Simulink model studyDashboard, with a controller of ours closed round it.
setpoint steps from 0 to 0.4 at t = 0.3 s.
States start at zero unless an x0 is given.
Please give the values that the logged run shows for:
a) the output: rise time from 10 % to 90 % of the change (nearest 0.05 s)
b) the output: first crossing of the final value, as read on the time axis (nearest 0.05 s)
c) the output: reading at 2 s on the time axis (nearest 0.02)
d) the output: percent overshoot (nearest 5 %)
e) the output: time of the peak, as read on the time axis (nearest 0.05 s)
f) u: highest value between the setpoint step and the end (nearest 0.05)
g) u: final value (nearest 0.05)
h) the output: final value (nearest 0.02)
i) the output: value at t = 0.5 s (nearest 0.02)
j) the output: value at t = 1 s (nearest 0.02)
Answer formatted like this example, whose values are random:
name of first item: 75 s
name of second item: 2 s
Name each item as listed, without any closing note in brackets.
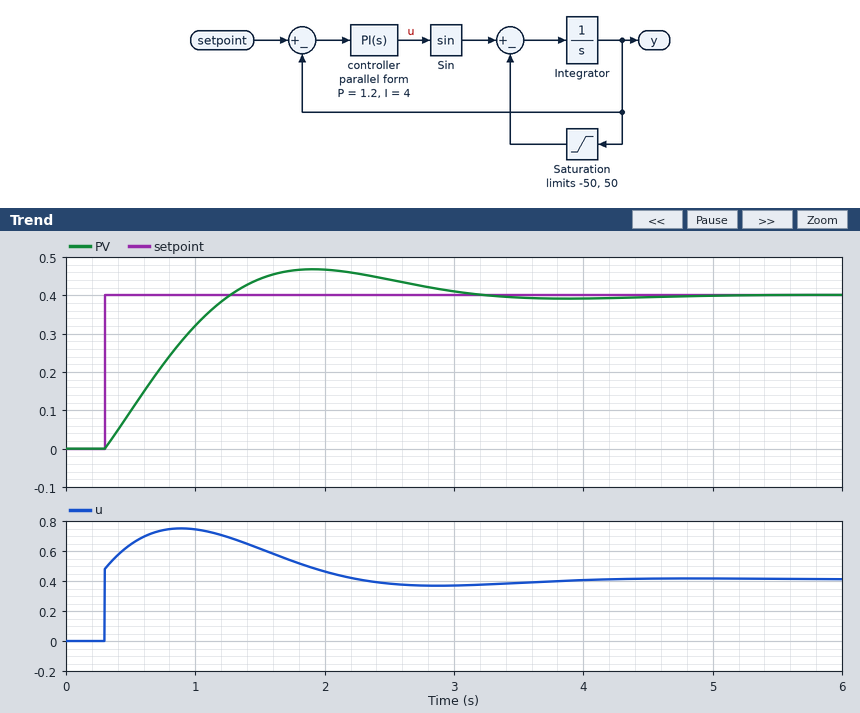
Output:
the output: rise time from 10 % to 90 % of the change: 0.75 s
the output: first crossing of the final value, as read on the time axis: 1.25 s
the output: reading at 2 s on the time axis: 0.46
the output: percent overshoot: 15 %
the output: time of the peak, as read on the time axis: 1.90 s
u: highest value between the setpoint step and the end: 0.75
u: final value: 0.40
the output: final value: 0.40
the output: value at t = 0.5 s: 0.10
the output: value at t = 1 s: 0.32
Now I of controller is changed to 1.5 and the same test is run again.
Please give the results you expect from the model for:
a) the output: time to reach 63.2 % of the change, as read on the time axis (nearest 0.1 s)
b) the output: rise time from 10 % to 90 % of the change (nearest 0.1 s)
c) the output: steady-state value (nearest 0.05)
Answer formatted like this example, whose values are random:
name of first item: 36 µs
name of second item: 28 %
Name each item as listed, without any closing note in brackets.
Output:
the output: time to reach 63.2 % of the change, as read on the time axis: 1.1 s
the output: rise time from 10 % to 90 % of the change: 1.5 s
the output: steady-state value: 0.40
